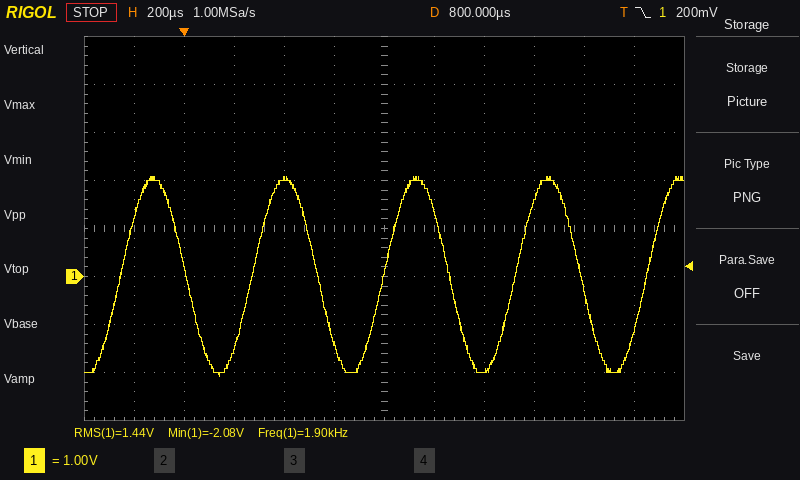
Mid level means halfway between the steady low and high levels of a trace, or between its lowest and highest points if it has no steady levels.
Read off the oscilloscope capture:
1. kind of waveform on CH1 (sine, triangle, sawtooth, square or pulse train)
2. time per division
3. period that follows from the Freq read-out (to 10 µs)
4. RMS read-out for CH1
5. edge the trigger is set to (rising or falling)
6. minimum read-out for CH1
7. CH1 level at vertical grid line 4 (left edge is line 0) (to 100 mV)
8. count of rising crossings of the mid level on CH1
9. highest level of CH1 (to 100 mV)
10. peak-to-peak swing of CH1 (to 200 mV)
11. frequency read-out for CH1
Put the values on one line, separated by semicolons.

sine; 200 µs; 530 µs; 1.44 V; falling; -2.08 V; 2.0 V; 5; 2.1 V; 4.2 V; 1.90 kHz
